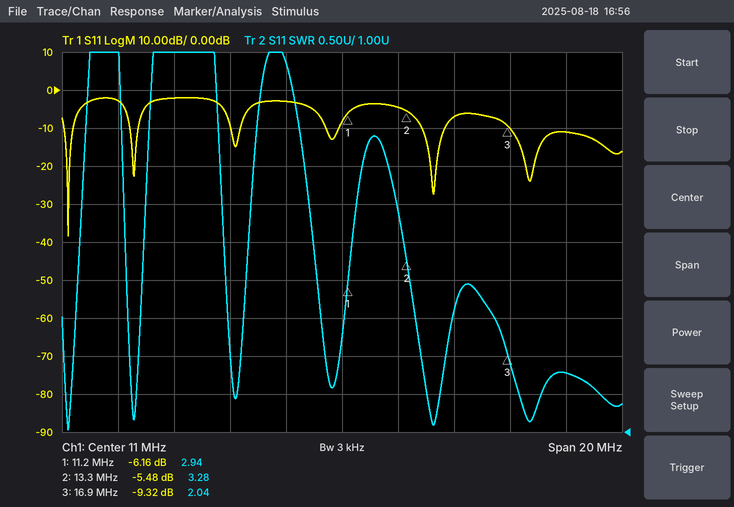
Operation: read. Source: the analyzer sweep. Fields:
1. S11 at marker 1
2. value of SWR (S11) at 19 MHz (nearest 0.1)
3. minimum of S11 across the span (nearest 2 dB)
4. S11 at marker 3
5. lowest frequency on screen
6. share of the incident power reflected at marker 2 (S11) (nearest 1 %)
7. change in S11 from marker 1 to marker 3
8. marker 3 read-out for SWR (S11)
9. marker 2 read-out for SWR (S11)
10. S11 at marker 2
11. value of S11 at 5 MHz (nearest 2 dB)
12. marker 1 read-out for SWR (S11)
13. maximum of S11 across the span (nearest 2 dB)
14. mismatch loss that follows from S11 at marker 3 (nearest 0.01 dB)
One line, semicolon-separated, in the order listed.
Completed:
-6.16 dB; 1.8; -38 dB; -9.32 dB; 1 MHz; 28 %; -3.16 dB; 2.04; 3.28; -5.48 dB; -2 dB; 2.94; -2 dB; 0.54 dB
